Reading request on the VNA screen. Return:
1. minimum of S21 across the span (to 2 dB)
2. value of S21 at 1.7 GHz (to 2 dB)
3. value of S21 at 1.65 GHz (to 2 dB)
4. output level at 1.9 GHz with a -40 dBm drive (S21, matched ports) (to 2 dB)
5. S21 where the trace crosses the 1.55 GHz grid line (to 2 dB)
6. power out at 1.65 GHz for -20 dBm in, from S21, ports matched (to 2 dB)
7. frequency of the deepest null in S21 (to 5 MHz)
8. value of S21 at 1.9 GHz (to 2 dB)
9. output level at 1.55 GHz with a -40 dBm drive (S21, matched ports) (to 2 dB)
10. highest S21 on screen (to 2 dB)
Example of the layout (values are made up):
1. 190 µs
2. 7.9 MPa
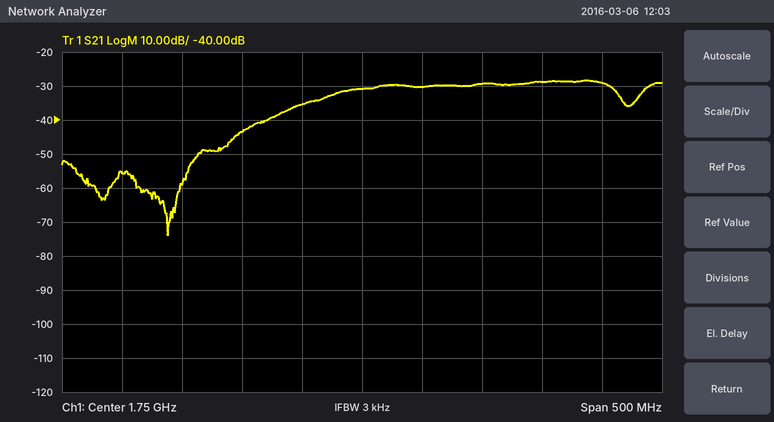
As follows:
1. -74 dB
2. -36 dB
3. -44 dB
4. -68 dBm
5. -56 dB
6. -64 dBm
7. 1.590 GHz
8. -28 dB
9. -96 dBm
10. -28 dB
